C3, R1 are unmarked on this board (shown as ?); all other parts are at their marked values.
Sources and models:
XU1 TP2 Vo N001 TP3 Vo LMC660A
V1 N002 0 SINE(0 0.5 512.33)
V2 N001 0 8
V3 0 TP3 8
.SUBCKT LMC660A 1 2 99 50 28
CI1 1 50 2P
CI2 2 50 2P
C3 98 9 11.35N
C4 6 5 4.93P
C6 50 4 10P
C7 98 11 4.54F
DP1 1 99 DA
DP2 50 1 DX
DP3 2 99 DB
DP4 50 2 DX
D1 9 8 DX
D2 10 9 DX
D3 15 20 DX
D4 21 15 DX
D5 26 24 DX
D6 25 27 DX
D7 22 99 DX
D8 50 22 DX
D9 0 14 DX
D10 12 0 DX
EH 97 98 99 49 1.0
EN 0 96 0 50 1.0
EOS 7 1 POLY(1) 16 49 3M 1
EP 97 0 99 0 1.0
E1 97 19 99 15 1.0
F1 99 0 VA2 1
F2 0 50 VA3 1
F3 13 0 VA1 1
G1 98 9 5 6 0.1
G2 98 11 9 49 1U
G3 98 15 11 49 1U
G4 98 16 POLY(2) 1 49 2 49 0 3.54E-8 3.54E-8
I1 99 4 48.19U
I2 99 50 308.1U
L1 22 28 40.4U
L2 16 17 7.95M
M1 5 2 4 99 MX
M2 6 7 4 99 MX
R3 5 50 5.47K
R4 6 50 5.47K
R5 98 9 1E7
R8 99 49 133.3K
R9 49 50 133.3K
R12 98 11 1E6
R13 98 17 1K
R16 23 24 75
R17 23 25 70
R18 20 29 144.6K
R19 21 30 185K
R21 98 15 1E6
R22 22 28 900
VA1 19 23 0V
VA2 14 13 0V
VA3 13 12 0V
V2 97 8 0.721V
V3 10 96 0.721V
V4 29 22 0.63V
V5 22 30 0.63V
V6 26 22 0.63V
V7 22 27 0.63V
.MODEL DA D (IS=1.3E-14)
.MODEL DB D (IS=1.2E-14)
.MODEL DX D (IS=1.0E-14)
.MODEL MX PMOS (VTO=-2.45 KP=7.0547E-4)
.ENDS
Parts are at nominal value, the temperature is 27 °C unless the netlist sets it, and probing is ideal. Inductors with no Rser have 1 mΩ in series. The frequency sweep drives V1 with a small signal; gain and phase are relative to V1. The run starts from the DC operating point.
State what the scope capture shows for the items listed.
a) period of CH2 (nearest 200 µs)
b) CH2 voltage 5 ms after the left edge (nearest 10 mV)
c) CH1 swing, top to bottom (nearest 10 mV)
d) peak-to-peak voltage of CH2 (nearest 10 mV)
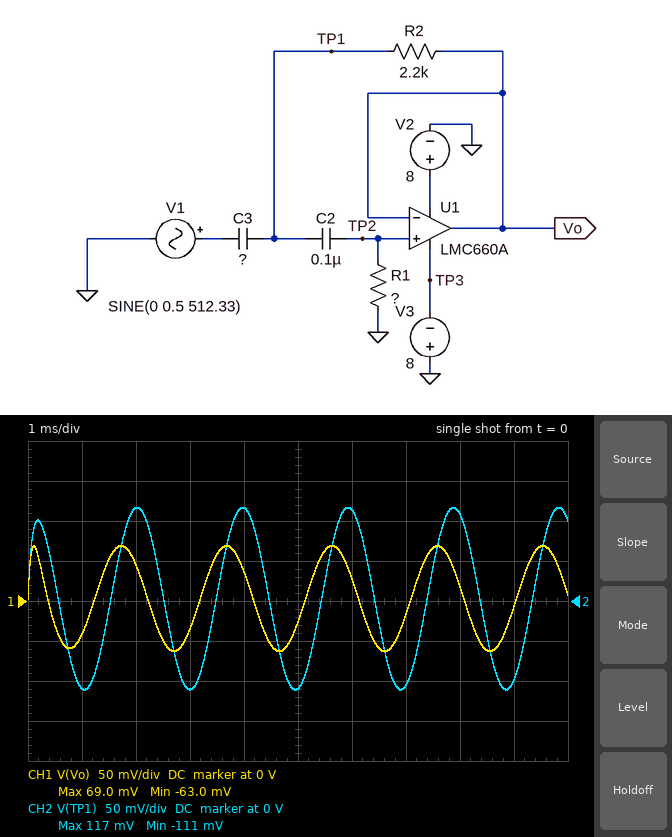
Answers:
2.0 ms
-110 mV
130 mV
230 mV
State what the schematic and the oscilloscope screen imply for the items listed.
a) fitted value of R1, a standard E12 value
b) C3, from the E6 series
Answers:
2.2 kΩ
33 nF
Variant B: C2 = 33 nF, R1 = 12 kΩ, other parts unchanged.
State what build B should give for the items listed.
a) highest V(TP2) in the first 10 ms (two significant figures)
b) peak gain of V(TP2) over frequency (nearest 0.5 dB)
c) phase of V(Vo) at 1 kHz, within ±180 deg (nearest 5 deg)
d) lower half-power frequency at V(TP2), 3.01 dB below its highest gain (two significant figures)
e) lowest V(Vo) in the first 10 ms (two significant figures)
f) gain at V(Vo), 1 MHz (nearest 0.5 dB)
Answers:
180 mV
2.0 dB
80 deg
790 Hz
-200 mV
-0.5 dB
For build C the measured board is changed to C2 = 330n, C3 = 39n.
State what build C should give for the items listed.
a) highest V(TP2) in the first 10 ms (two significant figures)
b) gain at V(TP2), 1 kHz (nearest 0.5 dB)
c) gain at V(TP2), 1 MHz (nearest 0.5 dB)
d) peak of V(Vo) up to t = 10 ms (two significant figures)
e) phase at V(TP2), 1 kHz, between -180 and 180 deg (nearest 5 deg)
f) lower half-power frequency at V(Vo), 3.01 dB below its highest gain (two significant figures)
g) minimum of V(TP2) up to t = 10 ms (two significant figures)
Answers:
120 mV
-6.5 dB
0 dB
130 mV
75 deg
1.9 kHz
-120 mV
